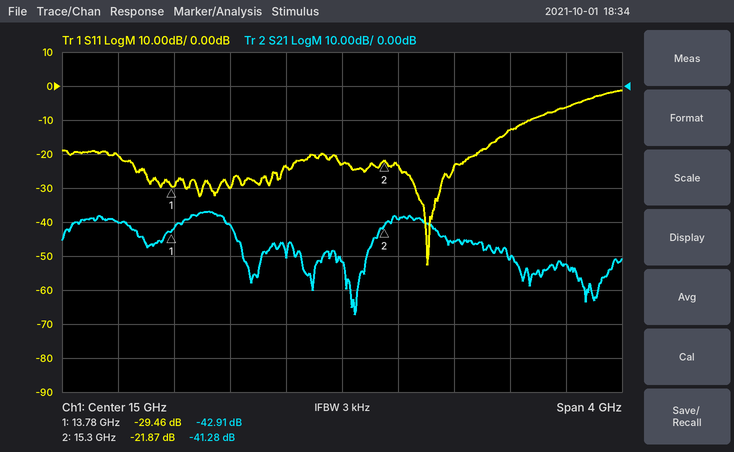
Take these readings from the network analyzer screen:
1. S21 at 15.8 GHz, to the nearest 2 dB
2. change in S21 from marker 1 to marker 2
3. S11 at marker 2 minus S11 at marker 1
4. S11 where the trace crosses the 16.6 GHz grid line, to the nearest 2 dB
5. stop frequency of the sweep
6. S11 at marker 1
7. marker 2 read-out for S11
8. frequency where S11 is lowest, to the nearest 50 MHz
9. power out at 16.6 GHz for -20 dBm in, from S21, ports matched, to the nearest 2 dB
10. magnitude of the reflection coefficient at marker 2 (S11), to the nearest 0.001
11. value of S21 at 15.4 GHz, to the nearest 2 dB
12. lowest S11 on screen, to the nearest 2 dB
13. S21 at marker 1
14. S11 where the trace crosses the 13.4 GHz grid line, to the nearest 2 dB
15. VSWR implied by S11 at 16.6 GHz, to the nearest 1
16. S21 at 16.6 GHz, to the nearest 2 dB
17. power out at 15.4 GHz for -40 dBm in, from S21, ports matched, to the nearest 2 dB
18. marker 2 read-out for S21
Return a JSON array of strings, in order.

["-46 dB", "1.63 dB", "7.59 dB", "-6 dB", "17 GHz", "-29.46 dB", "-21.87 dB", "15.60 GHz", "-72 dBm", "0.081", "-40 dB", "-52 dB", "-42.91 dB", "-20 dB", "3", "-52 dB", "-80 dBm", "-41.28 dB"]
